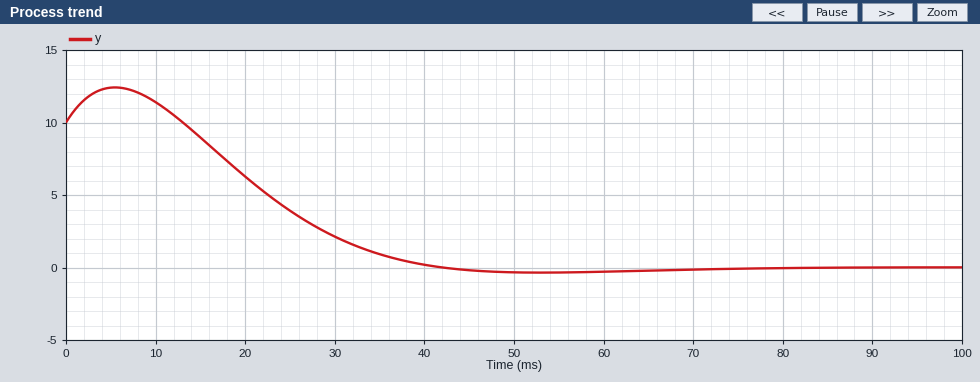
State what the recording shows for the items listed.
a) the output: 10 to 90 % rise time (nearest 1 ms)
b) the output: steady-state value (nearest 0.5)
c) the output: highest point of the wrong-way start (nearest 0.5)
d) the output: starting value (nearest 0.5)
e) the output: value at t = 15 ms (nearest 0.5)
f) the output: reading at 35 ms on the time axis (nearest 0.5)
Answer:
20 ms
0.0
12.5
10.0
9.0
1.0
